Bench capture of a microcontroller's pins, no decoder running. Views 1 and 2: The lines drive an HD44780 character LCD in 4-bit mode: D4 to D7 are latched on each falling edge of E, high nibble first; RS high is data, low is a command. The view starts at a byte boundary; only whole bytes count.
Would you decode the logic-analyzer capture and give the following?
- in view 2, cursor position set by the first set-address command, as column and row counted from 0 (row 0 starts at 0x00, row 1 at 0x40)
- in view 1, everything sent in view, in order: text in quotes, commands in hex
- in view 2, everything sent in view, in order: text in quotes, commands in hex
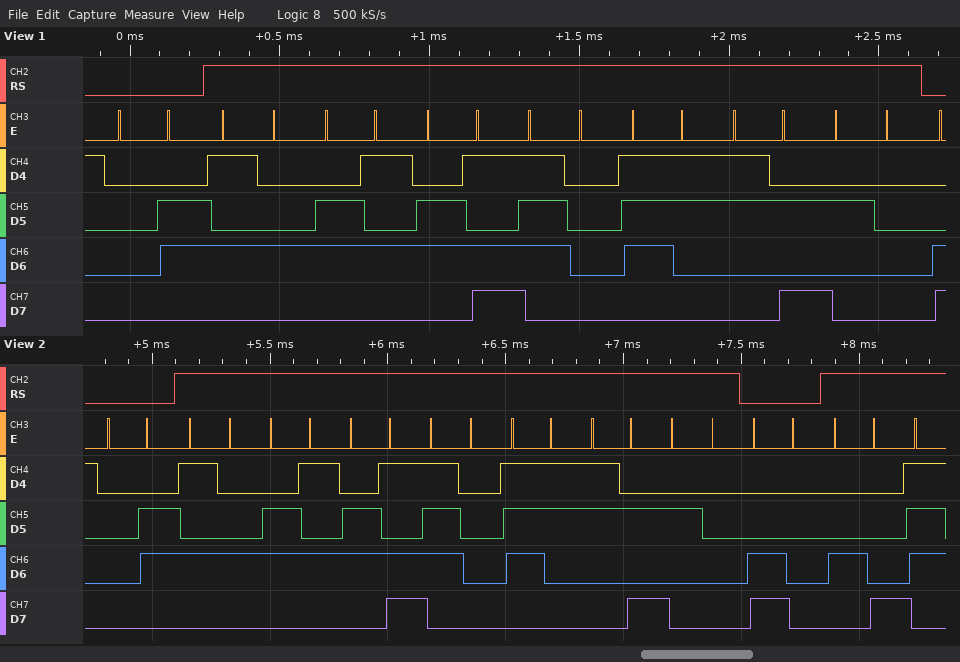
column 0, row 1
0x06 "Temps: "
0x06 "Temps: " 0xC0 "H"
